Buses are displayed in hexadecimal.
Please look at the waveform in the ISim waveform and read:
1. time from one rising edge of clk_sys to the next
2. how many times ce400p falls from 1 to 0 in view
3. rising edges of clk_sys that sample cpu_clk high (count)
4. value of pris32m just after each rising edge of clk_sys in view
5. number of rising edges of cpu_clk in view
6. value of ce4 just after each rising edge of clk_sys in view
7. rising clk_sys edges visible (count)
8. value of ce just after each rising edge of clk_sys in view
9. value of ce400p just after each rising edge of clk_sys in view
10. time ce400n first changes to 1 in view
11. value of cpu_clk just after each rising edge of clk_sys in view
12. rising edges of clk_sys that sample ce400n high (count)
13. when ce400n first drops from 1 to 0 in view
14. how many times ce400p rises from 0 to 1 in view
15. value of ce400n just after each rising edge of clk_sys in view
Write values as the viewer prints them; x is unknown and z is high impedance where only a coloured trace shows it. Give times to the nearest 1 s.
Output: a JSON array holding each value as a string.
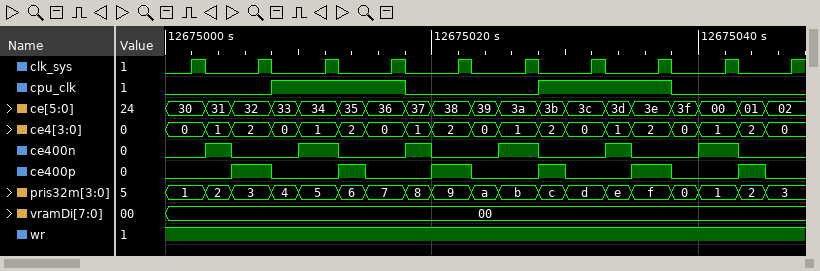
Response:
["5 s", "6", "4", "1, 3, 5, 7, 9, b, d, f, 1, 3", "2", "0, 2, 1, 0, 2, 1, 0, 2, 1, 0", "10", "30, 32, 34, 36, 38, 3a, 3c, 3e, 00, 02", "0 1 0 0 1 0 0 1 0 0", "12675003 s", "0 0 1 1 0 0 1 1 0 0", "3", "12675005 s", "6", "0 0 1 0 0 1 0 0 1 0"]
